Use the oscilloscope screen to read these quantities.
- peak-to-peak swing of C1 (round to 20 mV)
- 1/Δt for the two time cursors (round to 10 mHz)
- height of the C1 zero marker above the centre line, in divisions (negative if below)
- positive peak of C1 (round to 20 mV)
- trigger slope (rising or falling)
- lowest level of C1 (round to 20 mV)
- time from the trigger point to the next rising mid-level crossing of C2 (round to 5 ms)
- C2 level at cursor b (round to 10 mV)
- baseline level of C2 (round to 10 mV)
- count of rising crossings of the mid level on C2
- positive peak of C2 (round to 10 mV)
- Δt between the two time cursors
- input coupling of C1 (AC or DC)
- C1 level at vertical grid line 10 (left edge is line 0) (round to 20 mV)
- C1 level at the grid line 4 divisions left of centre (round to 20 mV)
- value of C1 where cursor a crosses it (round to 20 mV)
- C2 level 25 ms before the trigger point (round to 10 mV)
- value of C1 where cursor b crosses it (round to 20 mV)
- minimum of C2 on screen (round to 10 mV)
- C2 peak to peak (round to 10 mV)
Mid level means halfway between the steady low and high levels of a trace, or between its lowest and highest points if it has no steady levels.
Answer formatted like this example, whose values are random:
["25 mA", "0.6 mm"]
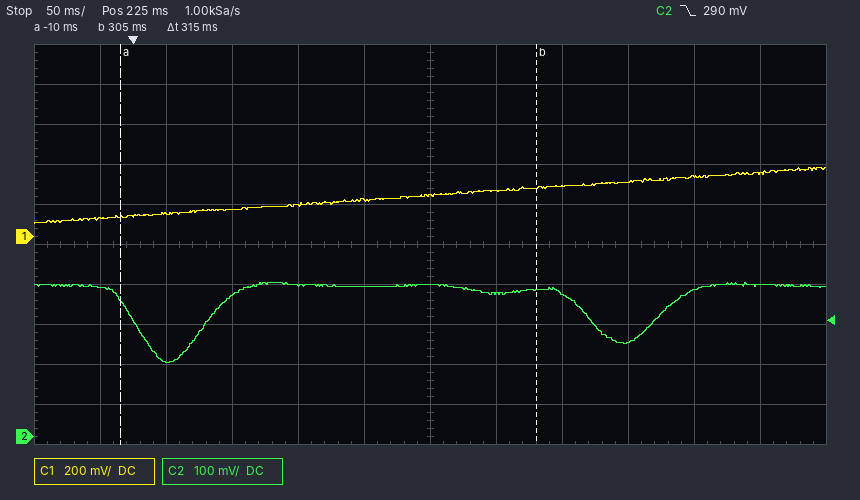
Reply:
["280 mV", "3.17 Hz", "+0.2 div", "340 mV", "falling", "60 mV", "55 ms", "370 mV", "380 mV", "2", "380 mV", "315 ms", "DC", "300 mV", "120 mV", "100 mV", "370 mV", "240 mV", "180 mV", "200 mV"]
